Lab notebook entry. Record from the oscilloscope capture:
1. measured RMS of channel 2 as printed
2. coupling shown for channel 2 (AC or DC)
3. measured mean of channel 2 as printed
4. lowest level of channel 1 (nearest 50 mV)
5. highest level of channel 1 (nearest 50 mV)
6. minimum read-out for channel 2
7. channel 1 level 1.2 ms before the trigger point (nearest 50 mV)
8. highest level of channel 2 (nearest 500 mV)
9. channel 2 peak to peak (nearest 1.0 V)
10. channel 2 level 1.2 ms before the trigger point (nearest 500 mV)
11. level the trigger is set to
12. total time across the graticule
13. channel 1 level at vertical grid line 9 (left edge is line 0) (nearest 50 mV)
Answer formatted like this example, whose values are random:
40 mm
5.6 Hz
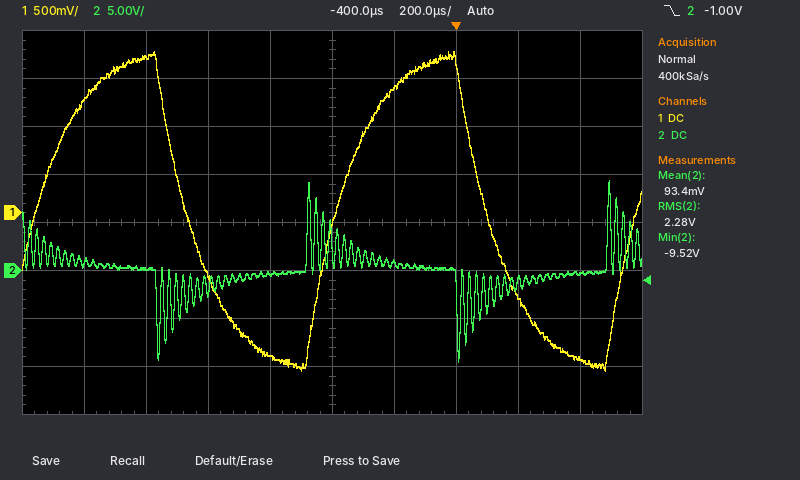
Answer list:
2.28 V
DC
93.4 mV
-1.65 V
1.70 V
-9.52 V
1.15 V
9.5 V
19.0 V
1.0 V
-1.00 V
2 ms
-1.50 V
